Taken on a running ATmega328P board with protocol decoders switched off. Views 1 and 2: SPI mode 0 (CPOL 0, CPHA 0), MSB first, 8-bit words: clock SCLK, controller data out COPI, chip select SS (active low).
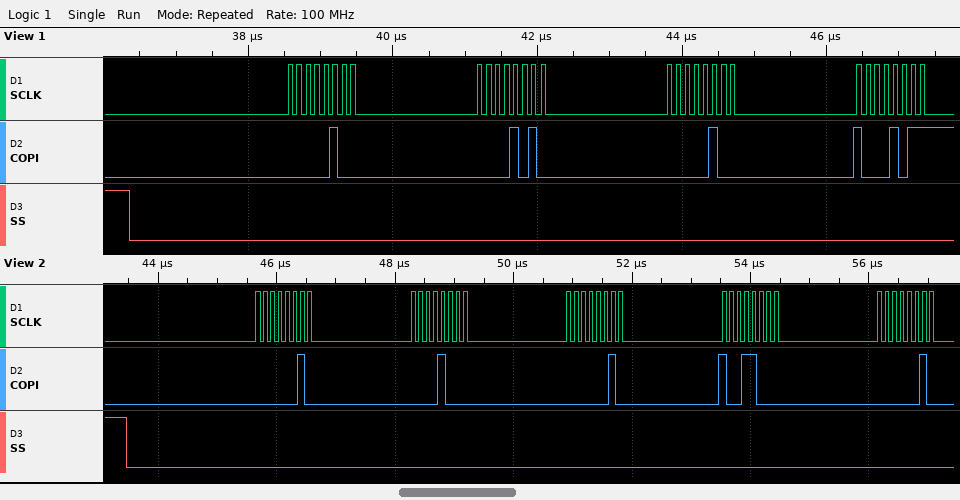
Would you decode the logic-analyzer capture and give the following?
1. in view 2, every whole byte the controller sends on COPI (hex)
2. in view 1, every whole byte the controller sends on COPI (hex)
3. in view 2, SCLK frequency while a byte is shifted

0x02 0x08 0x02 0x98 0x02
04 0A 04 8B
8 MHz
